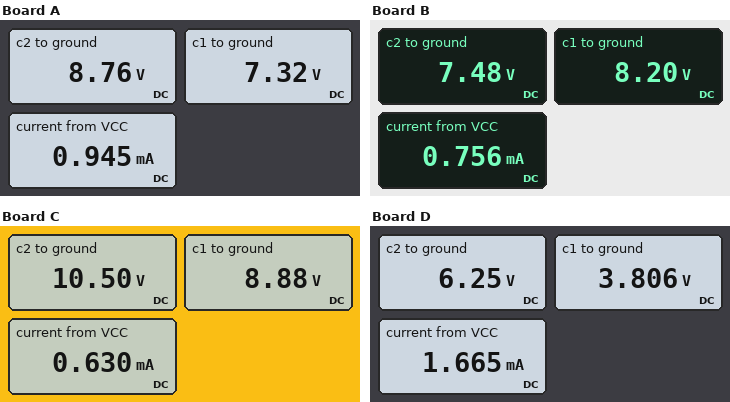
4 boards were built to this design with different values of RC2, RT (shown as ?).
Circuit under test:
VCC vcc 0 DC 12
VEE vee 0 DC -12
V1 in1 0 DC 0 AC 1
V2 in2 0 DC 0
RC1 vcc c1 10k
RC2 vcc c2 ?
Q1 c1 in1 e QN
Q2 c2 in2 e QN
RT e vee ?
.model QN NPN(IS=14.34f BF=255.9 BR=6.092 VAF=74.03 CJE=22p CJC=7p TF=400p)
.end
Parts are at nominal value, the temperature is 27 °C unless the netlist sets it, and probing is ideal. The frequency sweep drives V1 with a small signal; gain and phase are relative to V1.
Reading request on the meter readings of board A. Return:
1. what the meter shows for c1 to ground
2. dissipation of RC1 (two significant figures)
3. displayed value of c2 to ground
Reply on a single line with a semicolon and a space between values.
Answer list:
7.32 V; 2.2 mW; 8.76 V
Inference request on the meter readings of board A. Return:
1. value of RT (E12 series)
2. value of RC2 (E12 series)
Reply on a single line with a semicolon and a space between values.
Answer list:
12 kΩ; 6.8 kΩ
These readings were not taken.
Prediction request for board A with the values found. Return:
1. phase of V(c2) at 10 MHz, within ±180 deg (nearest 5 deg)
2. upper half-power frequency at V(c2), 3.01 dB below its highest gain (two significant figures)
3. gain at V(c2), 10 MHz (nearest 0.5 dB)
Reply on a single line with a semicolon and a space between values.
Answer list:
-50 deg; 8.2 MHz; 31.5 dB
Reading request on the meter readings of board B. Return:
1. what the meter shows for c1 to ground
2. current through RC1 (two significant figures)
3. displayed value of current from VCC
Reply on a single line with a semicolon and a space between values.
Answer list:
8.20 V; 380 µA; 0.756 mA
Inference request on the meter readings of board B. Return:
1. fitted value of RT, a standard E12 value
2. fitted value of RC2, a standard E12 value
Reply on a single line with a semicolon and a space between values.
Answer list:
15 kΩ; 12 kΩ
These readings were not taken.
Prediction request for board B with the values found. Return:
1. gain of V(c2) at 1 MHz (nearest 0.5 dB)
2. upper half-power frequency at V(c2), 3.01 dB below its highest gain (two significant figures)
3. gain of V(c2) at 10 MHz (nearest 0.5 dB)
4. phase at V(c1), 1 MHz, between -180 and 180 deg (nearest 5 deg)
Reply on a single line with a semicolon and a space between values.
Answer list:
38.0 dB; 4.4 MHz; 30.5 dB; 170 deg
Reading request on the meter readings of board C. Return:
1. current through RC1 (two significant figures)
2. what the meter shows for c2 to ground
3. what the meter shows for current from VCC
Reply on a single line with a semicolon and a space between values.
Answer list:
310 µA; 10.50 V; 0.630 mA
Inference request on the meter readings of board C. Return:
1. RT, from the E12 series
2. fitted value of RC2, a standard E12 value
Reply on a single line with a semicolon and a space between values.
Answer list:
18 kΩ; 4.7 kΩ
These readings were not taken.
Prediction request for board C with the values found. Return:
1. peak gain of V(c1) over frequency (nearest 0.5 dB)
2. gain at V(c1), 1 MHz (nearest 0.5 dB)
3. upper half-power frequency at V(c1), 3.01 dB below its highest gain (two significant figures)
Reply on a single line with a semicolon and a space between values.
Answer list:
35.5 dB; 35.5 dB; 5.4 MHz
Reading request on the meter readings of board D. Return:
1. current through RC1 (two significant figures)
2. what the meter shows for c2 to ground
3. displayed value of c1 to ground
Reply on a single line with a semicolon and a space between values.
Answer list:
820 µA; 6.25 V; 3.806 V
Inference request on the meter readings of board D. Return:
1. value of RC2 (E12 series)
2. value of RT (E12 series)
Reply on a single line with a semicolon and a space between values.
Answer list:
6.8 kΩ; 6.8 kΩ
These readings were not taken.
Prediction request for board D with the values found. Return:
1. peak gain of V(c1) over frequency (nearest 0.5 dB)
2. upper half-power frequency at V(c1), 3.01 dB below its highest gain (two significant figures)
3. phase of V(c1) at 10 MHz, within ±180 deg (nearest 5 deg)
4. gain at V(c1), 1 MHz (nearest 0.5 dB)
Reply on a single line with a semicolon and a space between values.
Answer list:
43.5 dB; 4.4 MHz; 115 deg; 43.0 dB
